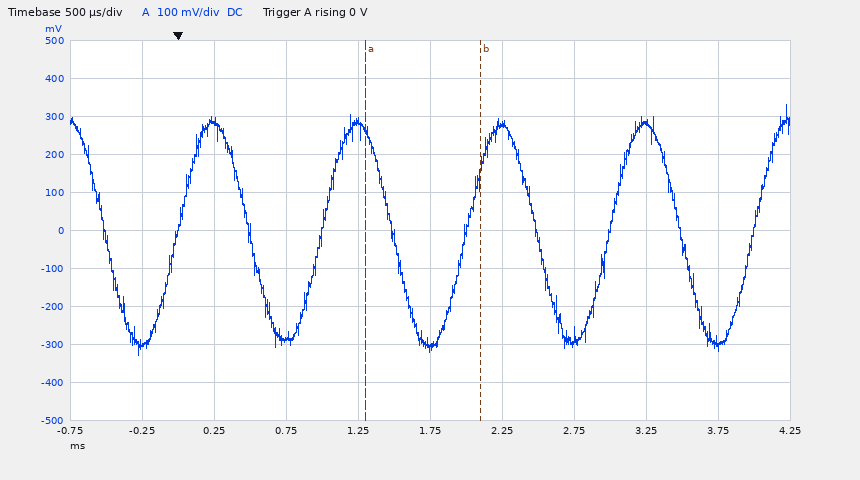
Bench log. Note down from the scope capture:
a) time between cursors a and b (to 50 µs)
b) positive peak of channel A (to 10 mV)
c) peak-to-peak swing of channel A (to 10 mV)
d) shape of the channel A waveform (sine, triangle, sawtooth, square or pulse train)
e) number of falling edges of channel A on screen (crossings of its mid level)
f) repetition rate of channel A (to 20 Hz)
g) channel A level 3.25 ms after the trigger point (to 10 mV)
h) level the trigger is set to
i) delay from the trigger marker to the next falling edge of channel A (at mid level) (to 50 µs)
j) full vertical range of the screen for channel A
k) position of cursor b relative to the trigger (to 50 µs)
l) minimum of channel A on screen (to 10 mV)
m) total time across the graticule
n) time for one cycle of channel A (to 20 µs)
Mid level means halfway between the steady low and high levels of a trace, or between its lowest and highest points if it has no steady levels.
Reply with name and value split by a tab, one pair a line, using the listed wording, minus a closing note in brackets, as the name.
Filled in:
time between cursors a and b	800 µs
positive peak of channel A	330 mV
peak-to-peak swing of channel A	660 mV
shape of the channel A waveform	sine
number of falling edges of channel A on screen	5
repetition rate of channel A	1.00 kHz
channel A level 3.25 ms after the trigger point	280 mV
level the trigger is set to	0 V
delay from the trigger marker to the next falling edge of channel A (at mid level)	500 µs
full vertical range of the screen for channel A	1 V
position of cursor b relative to the trigger	+2.10 ms
minimum of channel A on screen	-330 mV
total time across the graticule	5 ms
time for one cycle of channel A	1.00 ms
